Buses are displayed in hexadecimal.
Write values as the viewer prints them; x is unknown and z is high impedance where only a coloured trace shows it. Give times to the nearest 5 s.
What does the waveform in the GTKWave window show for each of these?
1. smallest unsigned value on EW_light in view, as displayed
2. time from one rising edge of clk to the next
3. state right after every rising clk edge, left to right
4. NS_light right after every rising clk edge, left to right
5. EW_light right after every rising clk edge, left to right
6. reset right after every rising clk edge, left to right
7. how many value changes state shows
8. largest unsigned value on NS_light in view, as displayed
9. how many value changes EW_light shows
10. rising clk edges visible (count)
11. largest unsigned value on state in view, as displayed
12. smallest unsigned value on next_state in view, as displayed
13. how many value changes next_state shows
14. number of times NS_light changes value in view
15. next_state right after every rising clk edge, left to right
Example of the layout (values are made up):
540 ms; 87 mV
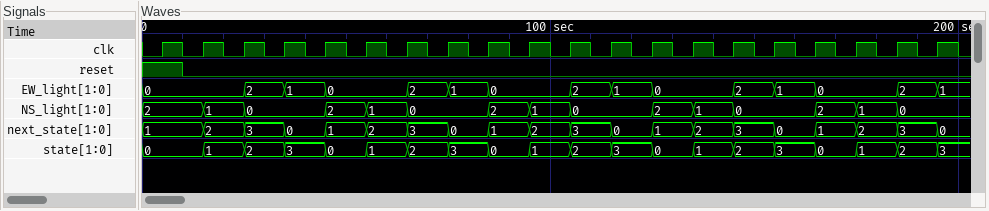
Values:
0; 10 s; 0, 1, 2, 3, 0, 1, 2, 3, 0, 1, 2, 3, 0, 1, 2, 3, 0, 1, 2, 3; 2, 1, 0, 0, 2, 1, 0, 0, 2, 1, 0, 0, 2, 1, 0, 0, 2, 1, 0, 0; 0, 0, 2, 1, 0, 0, 2, 1, 0, 0, 2, 1, 0, 0, 2, 1, 0, 0, 2, 1; 1 0 0 0 0 0 0 0 0 0 0 0 0 0 0 0 0 0 0 0; 19; 2; 14; 20; 3; 0; 19; 14; 1, 2, 3, 0, 1, 2, 3, 0, 1, 2, 3, 0, 1, 2, 3, 0, 1, 2, 3, 0
